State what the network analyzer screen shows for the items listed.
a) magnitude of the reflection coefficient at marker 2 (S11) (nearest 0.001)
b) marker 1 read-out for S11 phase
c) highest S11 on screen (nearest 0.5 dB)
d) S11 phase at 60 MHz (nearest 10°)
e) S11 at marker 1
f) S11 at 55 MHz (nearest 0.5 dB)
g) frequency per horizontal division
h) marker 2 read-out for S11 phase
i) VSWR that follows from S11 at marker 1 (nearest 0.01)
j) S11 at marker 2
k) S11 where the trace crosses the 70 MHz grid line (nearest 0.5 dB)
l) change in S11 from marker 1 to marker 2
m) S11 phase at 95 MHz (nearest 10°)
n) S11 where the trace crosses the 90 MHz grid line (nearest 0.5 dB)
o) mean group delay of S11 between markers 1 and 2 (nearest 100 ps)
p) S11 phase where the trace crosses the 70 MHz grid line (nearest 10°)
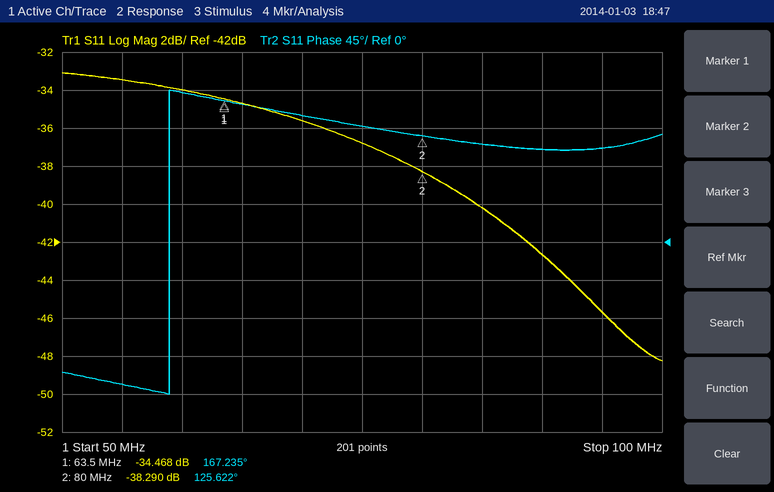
0.012
167.235°
-33.0 dB
180°
-34.468 dB
-33.5 dB
5 MHz
125.622°
1.04
-38.290 dB
-35.5 dB
-3.822 dB
110°
-42.5 dB
7.0 ns
150°
